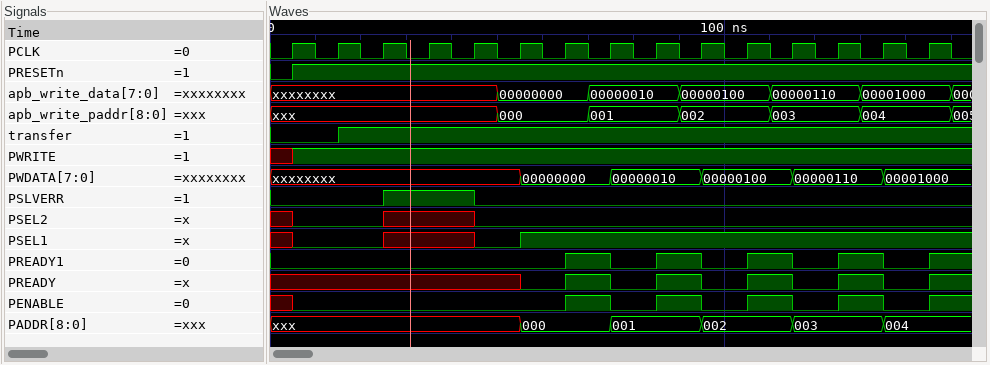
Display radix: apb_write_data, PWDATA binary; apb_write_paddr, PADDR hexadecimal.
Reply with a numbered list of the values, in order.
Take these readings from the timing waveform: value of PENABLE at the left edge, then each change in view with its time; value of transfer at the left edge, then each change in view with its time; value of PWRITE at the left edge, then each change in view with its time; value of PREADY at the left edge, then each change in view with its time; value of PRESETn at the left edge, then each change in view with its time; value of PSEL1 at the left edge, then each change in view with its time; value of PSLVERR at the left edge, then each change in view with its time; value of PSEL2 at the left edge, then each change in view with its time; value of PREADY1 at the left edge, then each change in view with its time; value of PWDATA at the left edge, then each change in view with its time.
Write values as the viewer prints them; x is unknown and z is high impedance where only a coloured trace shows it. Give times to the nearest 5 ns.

1. x, 0 at 5 ns, 1 at 65 ns, 0 at 75 ns, 1 at 85 ns, 0 at 95 ns, 1 at 105 ns, 0 at 115 ns, 1 at 125 ns, 0 at 135 ns, 1 at 145 ns
2. 0, 1 at 15 ns
3. x, 1 at 5 ns
4. x, 0 at 55 ns, 1 at 65 ns, 0 at 75 ns, 1 at 85 ns, 0 at 95 ns, 1 at 105 ns, 0 at 115 ns, 1 at 125 ns, 0 at 135 ns, 1 at 145 ns
5. 0, 1 at 5 ns
6. x, 0 at 5 ns, x at 25 ns, 0 at 45 ns, 1 at 55 ns
7. 0, 1 at 25 ns, 0 at 45 ns
8. x, 0 at 5 ns, x at 25 ns, 0 at 45 ns
9. 0, 1 at 65 ns, 0 at 75 ns, 1 at 85 ns, 0 at 95 ns, 1 at 105 ns, 0 at 115 ns, 1 at 125 ns, 0 at 135 ns, 1 at 145 ns
10. xxxxxxxx, 00000000 at 55 ns, 00000010 at 75 ns, 00000100 at 95 ns, 00000110 at 115 ns, 00001000 at 135 ns
